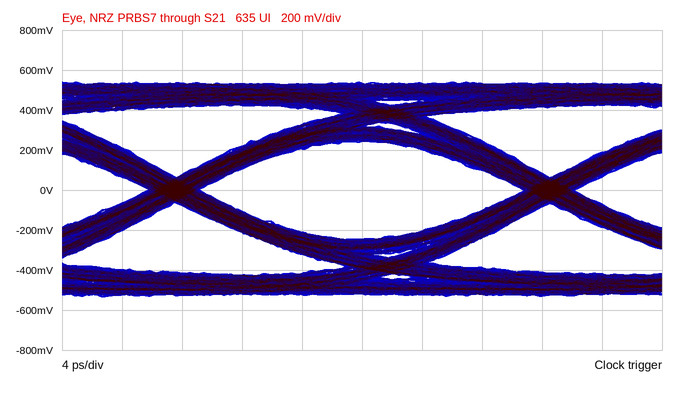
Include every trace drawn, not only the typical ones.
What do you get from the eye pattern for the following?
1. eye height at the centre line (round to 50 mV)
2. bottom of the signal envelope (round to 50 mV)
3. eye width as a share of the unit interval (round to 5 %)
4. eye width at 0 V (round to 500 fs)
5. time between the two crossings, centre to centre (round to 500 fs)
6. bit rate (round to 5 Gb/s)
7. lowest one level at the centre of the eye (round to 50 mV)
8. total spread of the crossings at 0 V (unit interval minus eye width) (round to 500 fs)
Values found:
500 mV
-550 mV
85 %
21.5 ps
25.0 ps
40 Gb/s
250 mV
3.5 ps
